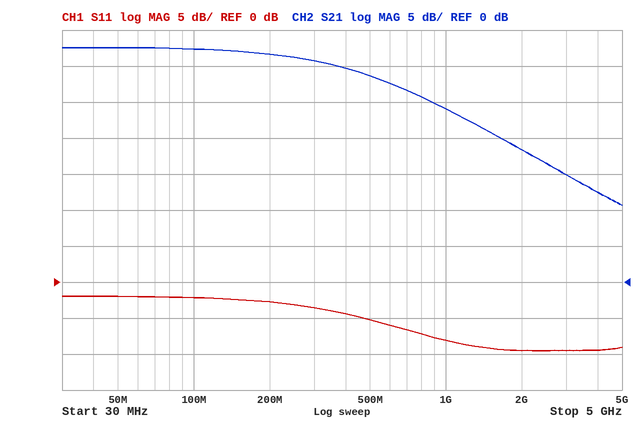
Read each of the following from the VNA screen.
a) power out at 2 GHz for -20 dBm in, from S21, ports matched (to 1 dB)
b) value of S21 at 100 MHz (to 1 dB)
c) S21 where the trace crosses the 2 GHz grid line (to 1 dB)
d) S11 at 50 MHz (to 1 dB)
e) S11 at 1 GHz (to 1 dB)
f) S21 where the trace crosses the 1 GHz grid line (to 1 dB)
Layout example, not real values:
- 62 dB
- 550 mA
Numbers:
- -2 dBm
- 32 dB
- 18 dB
- -2 dB
- -8 dB
- 24 dB
